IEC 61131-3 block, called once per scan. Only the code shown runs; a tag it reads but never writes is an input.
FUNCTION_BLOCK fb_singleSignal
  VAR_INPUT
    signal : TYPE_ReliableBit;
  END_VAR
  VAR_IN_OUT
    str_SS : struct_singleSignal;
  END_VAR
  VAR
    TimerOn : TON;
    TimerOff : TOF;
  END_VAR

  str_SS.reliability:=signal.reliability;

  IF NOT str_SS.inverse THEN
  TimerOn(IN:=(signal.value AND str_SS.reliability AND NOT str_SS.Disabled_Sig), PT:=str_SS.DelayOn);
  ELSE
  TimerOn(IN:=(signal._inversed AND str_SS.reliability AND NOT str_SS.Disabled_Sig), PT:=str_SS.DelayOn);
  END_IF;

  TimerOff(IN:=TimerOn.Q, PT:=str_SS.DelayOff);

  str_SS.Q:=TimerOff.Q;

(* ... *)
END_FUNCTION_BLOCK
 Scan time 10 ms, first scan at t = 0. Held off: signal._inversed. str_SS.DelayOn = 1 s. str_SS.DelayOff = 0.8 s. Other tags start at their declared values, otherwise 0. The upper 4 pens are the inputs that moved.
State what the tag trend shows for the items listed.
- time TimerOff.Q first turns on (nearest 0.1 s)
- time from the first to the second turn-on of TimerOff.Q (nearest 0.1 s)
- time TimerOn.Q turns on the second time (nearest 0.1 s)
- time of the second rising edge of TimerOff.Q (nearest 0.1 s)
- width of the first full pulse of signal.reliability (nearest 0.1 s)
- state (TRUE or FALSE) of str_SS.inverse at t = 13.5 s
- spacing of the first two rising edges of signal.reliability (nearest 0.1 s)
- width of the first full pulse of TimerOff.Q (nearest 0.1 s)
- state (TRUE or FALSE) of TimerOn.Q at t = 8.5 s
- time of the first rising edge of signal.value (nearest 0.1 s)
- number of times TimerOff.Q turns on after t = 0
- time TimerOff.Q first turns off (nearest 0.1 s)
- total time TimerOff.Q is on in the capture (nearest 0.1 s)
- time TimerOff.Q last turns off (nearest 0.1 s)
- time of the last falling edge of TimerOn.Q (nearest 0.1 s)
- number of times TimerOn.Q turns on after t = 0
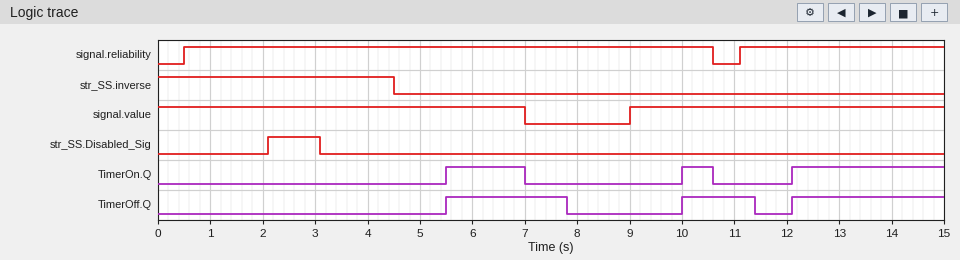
5.5 s
4.5 s
10.0 s
10.0 s
10.1 s
FALSE
10.6 s
2.3 s
FALSE
9.0 s
3
7.8 s
6.6 s
11.4 s
10.6 s
3
